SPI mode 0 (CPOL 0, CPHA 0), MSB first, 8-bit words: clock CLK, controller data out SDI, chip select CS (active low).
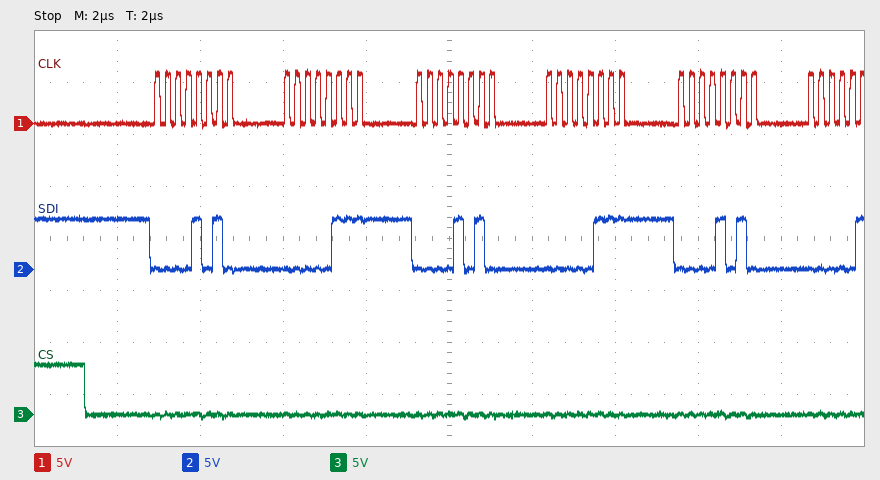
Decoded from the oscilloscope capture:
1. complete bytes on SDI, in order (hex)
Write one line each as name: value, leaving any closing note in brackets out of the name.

complete bytes on SDI, in order: 0A 07 0A 07 0A
